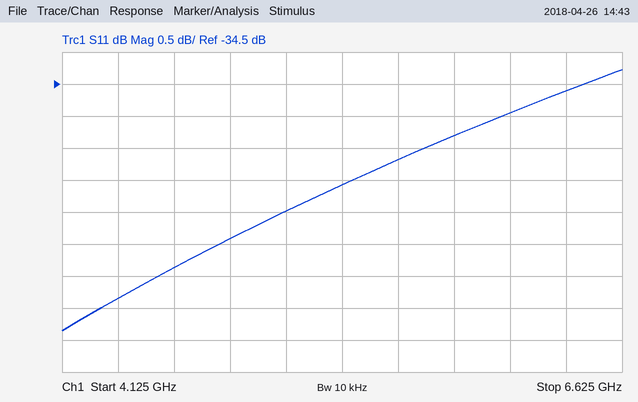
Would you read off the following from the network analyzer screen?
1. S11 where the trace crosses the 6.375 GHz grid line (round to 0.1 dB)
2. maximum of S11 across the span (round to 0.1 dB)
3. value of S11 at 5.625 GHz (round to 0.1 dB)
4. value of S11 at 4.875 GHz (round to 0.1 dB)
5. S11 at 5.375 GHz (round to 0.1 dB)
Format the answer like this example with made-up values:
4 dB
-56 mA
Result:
-34.6 dB
-34.3 dB
-35.7 dB
-36.9 dB
-36.1 dB
